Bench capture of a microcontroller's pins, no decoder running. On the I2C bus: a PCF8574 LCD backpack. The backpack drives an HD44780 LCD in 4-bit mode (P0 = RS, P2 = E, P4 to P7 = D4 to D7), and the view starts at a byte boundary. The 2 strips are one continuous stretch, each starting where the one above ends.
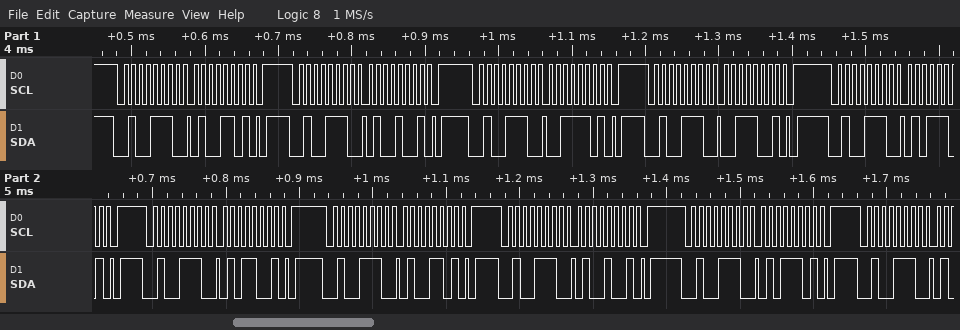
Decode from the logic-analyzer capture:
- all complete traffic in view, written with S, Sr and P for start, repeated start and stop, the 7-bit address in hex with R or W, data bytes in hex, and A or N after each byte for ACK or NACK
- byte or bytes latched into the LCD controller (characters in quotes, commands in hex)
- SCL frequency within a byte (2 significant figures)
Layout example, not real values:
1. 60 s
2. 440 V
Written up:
1. S 27W A 4D A P S 27W A 49 A P S 27W A 3D A P S 27W A 39 A P S 27W A 5D A P S 27W A 59 A P S 27W A 4D A P S 27W A 49 A P S 27W A 5D A P S 27W A
2. 'C' 'T'
3. 100 kHz
